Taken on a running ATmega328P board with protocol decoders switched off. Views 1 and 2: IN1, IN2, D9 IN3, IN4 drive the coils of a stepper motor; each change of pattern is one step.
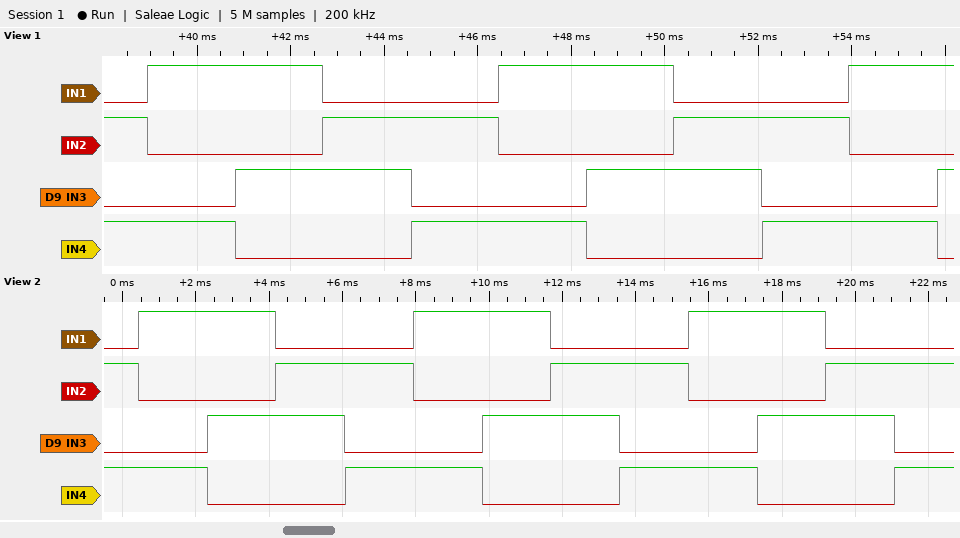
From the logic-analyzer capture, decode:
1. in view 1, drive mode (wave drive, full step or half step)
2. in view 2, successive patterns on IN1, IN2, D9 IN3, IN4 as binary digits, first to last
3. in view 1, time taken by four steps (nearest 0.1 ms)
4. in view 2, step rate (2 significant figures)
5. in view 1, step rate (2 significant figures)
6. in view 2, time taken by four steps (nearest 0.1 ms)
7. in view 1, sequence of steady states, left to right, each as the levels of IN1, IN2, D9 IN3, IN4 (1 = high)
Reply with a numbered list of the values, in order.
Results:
1. full step
2. 0101 1001 1010 0110 0101 1001 1010 0110 0101 1001 1010 0110 0101
3. 7.5 ms
4. 530 steps/s
5. 530 steps/s
6. 7.5 ms
7. 0101 1001 1010 0110 0101 1001 1010 0110 0101 1001 1010
